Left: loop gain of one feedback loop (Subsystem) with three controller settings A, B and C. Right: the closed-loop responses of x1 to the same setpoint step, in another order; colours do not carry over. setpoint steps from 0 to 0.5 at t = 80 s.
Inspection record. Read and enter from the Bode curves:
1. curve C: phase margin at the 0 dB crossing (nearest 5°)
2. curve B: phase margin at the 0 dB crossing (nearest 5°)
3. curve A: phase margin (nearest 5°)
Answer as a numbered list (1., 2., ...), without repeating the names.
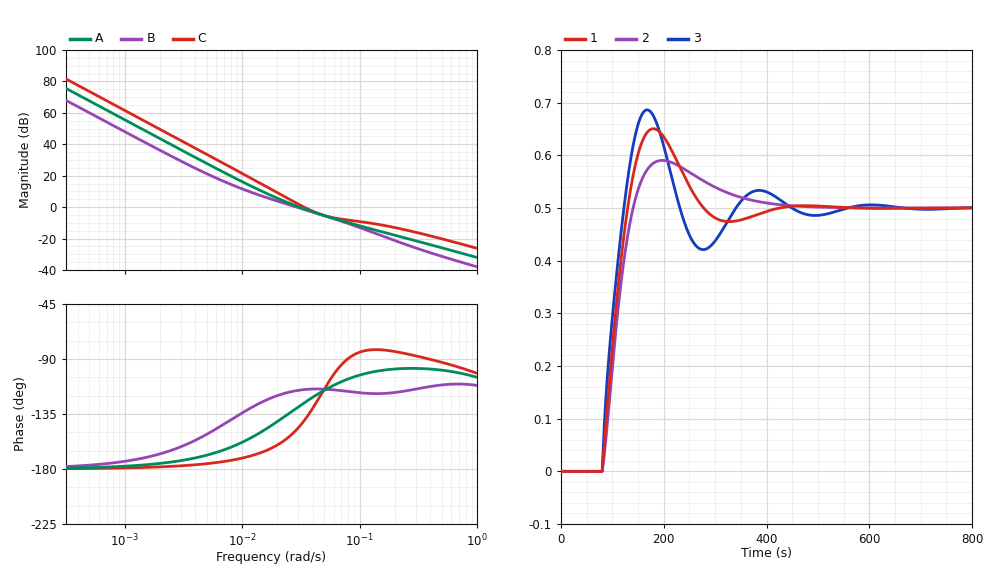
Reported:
1. 40°
2. 65°
3. 50°
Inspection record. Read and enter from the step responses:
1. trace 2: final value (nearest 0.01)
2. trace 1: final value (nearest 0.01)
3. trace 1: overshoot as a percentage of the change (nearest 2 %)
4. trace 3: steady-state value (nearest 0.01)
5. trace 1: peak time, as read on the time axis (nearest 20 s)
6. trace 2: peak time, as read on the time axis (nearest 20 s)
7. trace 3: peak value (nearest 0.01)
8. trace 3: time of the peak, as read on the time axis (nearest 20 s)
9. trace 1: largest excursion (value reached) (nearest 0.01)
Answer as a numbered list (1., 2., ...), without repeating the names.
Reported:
1. 0.50
2. 0.50
3. 30 %
4. 0.50
5. 180 s
6. 200 s
7. 0.69
8. 160 s
9. 0.65
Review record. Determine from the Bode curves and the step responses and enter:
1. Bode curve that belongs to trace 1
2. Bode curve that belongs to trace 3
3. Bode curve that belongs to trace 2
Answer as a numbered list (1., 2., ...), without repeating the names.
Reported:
1. A
2. C
3. B
